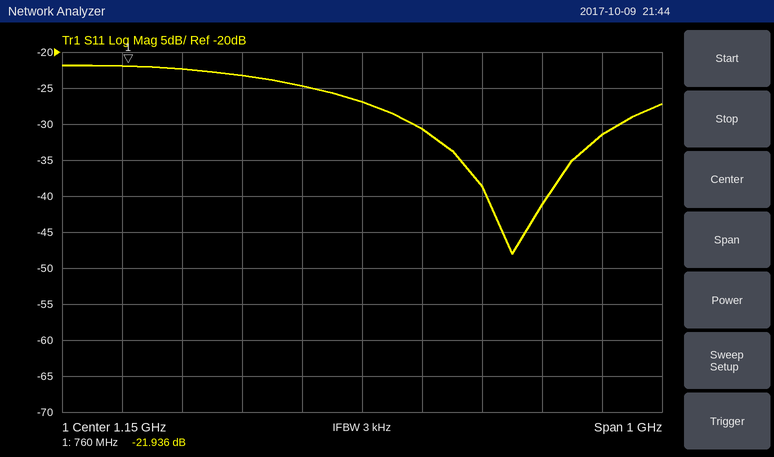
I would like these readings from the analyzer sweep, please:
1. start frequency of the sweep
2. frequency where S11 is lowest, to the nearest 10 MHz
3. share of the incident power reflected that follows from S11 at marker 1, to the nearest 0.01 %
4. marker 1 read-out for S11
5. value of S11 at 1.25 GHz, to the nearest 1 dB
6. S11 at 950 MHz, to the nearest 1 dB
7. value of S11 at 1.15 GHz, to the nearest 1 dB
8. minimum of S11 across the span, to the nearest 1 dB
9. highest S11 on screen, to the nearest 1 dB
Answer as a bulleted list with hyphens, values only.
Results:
- 650 MHz
- 1.40 GHz
- 0.64 %
- -21.936 dB
- -31 dB
- -23 dB
- -27 dB
- -48 dB
- -22 dB
